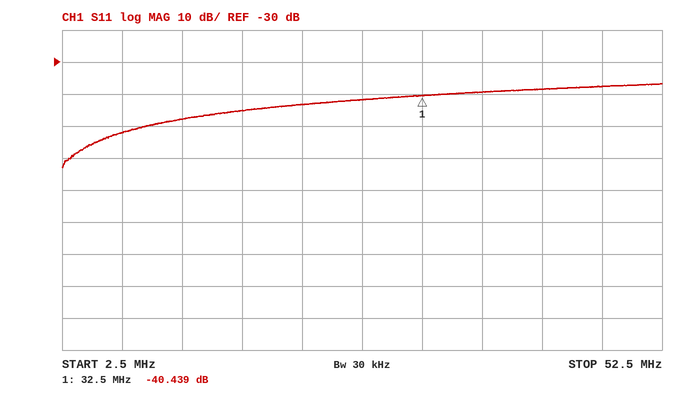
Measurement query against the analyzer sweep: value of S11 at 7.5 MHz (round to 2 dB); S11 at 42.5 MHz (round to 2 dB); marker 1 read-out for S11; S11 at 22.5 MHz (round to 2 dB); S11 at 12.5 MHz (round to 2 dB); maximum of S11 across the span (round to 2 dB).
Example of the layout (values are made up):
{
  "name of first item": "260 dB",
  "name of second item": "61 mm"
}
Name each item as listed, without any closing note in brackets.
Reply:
{
  "value of S11 at 7.5 MHz": "-52 dB",
  "S11 at 42.5 MHz": "-38 dB",
  "marker 1 read-out for S11": "-40.439 dB",
  "S11 at 22.5 MHz": "-44 dB",
  "S11 at 12.5 MHz": "-48 dB",
  "maximum of S11 across the span": "-36 dB"
}
